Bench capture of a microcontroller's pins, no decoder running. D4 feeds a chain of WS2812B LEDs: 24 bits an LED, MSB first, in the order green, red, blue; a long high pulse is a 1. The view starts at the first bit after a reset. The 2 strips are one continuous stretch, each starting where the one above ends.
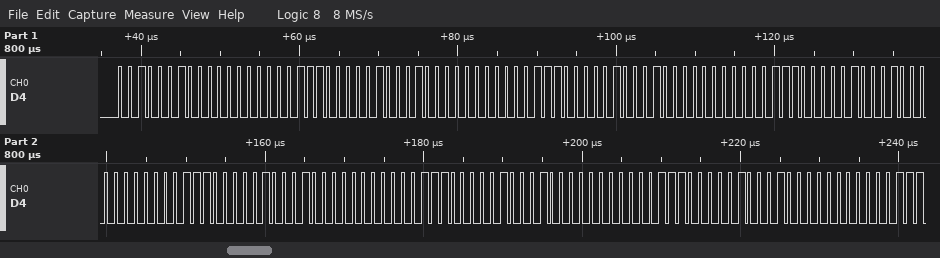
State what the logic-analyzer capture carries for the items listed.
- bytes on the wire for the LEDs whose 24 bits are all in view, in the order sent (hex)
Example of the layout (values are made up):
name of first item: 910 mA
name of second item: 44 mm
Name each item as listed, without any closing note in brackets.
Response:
bytes on the wire for the LEDs whose 24 bits are all in view, in the order sent: 22 00 38 22 00 38 22 00 38 22 00 38 22 00 38 22 00 38
